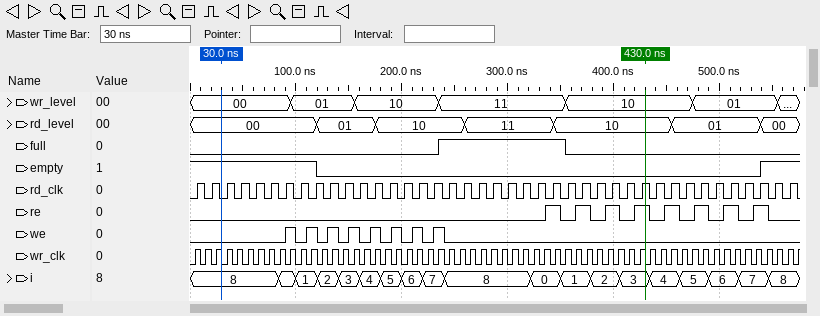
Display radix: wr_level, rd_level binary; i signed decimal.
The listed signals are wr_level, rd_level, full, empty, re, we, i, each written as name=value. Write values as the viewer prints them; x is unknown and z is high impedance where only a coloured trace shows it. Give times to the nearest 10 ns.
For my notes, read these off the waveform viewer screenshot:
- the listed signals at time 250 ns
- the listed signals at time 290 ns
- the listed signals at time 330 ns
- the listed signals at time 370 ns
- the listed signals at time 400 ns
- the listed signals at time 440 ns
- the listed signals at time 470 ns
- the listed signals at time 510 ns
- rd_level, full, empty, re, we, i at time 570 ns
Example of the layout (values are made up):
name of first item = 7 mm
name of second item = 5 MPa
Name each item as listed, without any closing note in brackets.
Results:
the listed signals at time 250 ns = wr_level=11, rd_level=10, full=1, empty=0, re=0, we=0, i=8
the listed signals at time 290 ns = wr_level=11, rd_level=11, full=1, empty=0, re=0, we=0, i=8
the listed signals at time 330 ns = wr_level=11, rd_level=11, full=1, empty=0, re=0, we=0, i=0
the listed signals at time 370 ns = wr_level=10, rd_level=10, full=0, empty=0, re=1, we=0, i=1
the listed signals at time 400 ns = wr_level=10, rd_level=10, full=0, empty=0, re=1, we=0, i=2
the listed signals at time 440 ns = wr_level=10, rd_level=10, full=0, empty=0, re=0, we=0, i=4
the listed signals at time 470 ns = wr_level=10, rd_level=01, full=0, empty=0, re=0, we=0, i=5
the listed signals at time 510 ns = wr_level=01, rd_level=01, full=0, empty=0, re=1, we=0, i=6
rd_level, full, empty, re, we, i at time 570 ns = rd_level=00, full=0, empty=1, re=0, we=0, i=8
